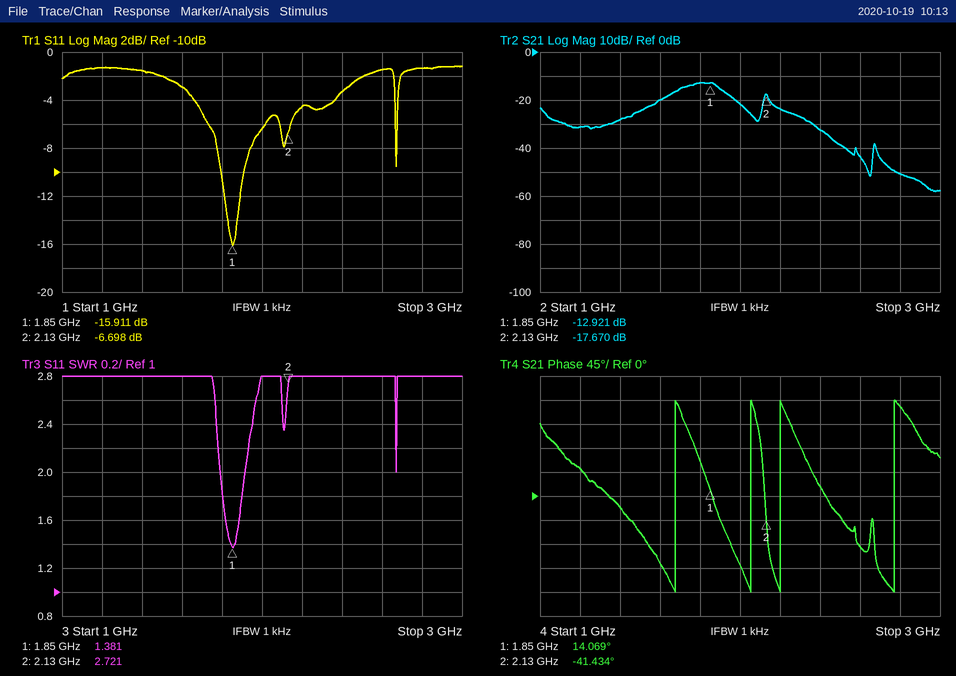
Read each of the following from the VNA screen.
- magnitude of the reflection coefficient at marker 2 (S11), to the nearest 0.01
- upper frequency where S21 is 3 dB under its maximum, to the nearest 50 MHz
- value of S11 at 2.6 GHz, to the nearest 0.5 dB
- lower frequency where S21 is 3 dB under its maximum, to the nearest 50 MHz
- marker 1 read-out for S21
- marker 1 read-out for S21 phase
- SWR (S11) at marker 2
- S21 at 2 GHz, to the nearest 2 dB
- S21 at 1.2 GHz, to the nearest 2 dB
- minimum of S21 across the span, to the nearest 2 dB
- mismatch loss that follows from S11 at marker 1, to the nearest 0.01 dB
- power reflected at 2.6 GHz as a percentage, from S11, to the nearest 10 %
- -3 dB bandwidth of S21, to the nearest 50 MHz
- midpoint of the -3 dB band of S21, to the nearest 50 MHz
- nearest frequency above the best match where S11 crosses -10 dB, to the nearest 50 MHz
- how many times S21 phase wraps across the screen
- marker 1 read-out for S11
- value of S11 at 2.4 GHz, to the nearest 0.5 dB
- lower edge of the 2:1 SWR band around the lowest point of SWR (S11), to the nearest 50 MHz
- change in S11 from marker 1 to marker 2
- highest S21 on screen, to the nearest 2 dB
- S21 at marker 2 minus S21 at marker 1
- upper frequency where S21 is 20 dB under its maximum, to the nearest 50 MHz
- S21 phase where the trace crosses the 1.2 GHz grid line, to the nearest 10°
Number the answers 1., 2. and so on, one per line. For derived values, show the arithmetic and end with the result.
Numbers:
1. 10^(-6.698/20) ≈ 0.46
2. 1.90 GHz
3. -1.5 dB
4. 1.70 GHz
5. -12.921 dB
6. 14.069°
7. 2.721
8. -22 dB
9. -32 dB
10. -58 dB
11. −10 log10(1 − 10^(-15.911/10)) ≈ 0.11 dB
12. 10^(-1.5/10) ≈ 70.8 %, so 70 % to the nearest 10 %
13. 1.90 GHz − 1.70 GHz = 200 MHz
14. 1.80 GHz
15. 1.90 GHz
16. 4
17. -15.911 dB
18. -3.5 dB
19. 1.80 GHz
20. -6.698 − (-15.911) = 9.213 dB
21. -12 dB
22. -17.67 − (-12.921) = -4.749 dB
23. 2.40 GHz
24. 50°
